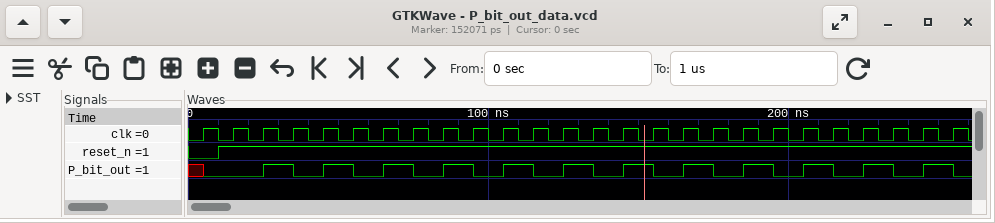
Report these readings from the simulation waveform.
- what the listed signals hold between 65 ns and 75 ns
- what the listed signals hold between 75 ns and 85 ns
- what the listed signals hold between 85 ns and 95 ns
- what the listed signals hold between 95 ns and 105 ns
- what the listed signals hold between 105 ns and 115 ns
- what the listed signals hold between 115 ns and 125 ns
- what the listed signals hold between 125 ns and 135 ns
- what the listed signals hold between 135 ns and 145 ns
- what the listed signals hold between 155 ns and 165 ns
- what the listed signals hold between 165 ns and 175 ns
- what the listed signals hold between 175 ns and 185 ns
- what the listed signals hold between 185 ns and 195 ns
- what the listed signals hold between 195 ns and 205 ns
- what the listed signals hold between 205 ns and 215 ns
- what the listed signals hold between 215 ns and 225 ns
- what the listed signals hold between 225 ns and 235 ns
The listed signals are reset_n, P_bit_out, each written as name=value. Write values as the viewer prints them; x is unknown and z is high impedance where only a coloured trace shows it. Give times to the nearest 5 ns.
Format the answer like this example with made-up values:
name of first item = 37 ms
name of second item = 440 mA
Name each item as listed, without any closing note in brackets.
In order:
what the listed signals hold between 65 ns and 75 ns = reset_n=1, P_bit_out=1
what the listed signals hold between 75 ns and 85 ns = reset_n=1, P_bit_out=0
what the listed signals hold between 85 ns and 95 ns = reset_n=1, P_bit_out=1
what the listed signals hold between 95 ns and 105 ns = reset_n=1, P_bit_out=0
what the listed signals hold between 105 ns and 115 ns = reset_n=1, P_bit_out=1
what the listed signals hold between 115 ns and 125 ns = reset_n=1, P_bit_out=0
what the listed signals hold between 125 ns and 135 ns = reset_n=1, P_bit_out=1
what the listed signals hold between 135 ns and 145 ns = reset_n=1, P_bit_out=0
what the listed signals hold between 155 ns and 165 ns = reset_n=1, P_bit_out=0
what the listed signals hold between 165 ns and 175 ns = reset_n=1, P_bit_out=1
what the listed signals hold between 175 ns and 185 ns = reset_n=1, P_bit_out=0
what the listed signals hold between 185 ns and 195 ns = reset_n=1, P_bit_out=1
what the listed signals hold between 195 ns and 205 ns = reset_n=1, P_bit_out=0
what the listed signals hold between 205 ns and 215 ns = reset_n=1, P_bit_out=1
what the listed signals hold between 215 ns and 225 ns = reset_n=1, P_bit_out=0
what the listed signals hold between 225 ns and 235 ns = reset_n=1, P_bit_out=1
